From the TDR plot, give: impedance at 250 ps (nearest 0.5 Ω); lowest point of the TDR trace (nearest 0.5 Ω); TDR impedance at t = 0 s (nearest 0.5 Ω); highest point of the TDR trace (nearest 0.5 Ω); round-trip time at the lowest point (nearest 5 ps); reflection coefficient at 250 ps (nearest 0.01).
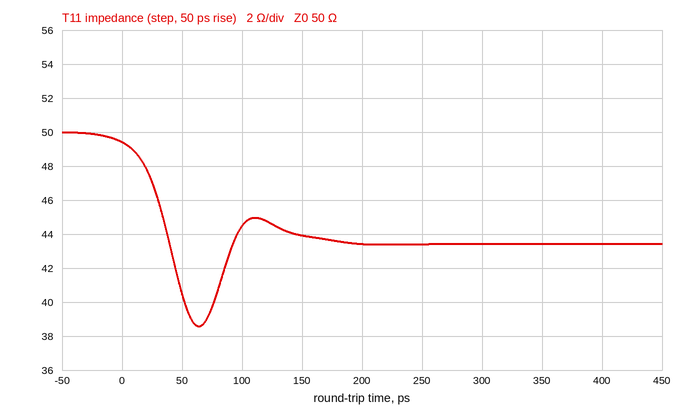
43.5 Ω
38.5 Ω
49.5 Ω
50.0 Ω
65 ps
-0.07
